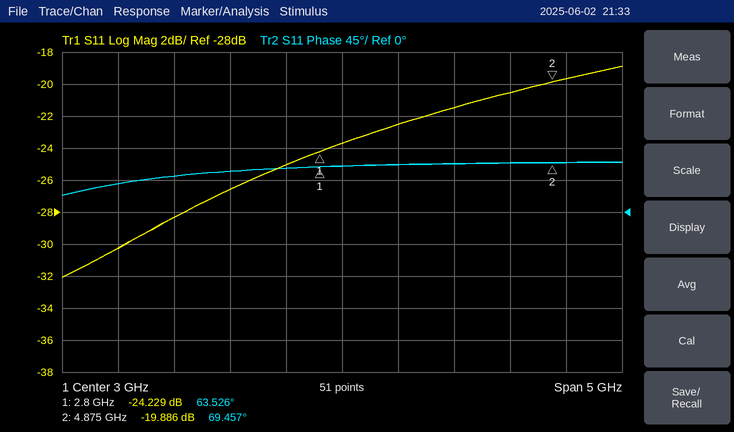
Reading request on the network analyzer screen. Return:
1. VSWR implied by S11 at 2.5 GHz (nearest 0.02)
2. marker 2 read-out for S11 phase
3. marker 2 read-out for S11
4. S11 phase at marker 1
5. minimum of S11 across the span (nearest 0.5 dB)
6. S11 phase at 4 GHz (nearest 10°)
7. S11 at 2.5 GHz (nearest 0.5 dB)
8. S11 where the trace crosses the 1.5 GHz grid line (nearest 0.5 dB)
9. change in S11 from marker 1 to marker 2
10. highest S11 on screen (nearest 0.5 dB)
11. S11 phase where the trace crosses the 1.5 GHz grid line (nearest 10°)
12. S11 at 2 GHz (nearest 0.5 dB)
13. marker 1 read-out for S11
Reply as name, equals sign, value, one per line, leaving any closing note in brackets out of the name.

VSWR implied by S11 at 2.5 GHz = 1.12
marker 2 read-out for S11 phase = 69.457°
marker 2 read-out for S11 = -19.886 dB
S11 phase at marker 1 = 63.526°
minimum of S11 across the span = -32.0 dB
S11 phase at 4 GHz = 70°
S11 at 2.5 GHz = -25.0 dB
S11 where the trace crosses the 1.5 GHz grid line = -28.5 dB
change in S11 from marker 1 to marker 2 = 4.343 dB
highest S11 on screen = -19.0 dB
S11 phase where the trace crosses the 1.5 GHz grid line = 50°
S11 at 2 GHz = -26.5 dB
marker 1 read-out for S11 = -24.229 dB
